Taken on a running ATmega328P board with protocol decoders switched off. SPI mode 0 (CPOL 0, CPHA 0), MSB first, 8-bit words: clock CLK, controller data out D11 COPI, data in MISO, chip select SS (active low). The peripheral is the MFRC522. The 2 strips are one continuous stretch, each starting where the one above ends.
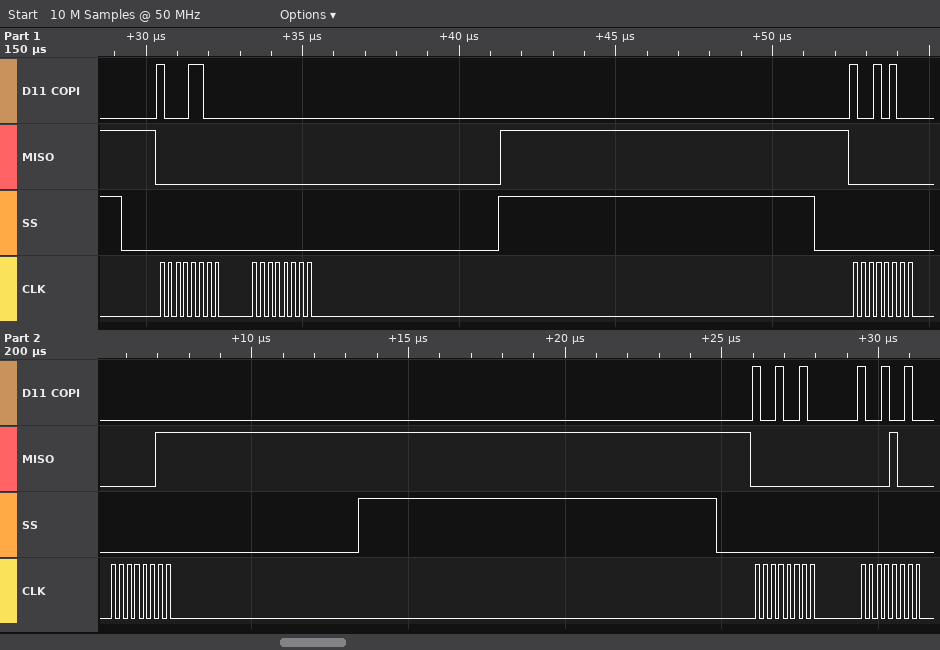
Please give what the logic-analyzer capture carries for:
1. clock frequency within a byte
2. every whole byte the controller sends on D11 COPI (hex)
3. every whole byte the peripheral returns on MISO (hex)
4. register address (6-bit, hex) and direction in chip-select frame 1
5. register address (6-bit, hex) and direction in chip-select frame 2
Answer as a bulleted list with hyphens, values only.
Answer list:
- 4 MHz
- 8C 00 94 00 92 92
- 00 00 00 03 00 08
- 0x06 read
- 0x0A read
